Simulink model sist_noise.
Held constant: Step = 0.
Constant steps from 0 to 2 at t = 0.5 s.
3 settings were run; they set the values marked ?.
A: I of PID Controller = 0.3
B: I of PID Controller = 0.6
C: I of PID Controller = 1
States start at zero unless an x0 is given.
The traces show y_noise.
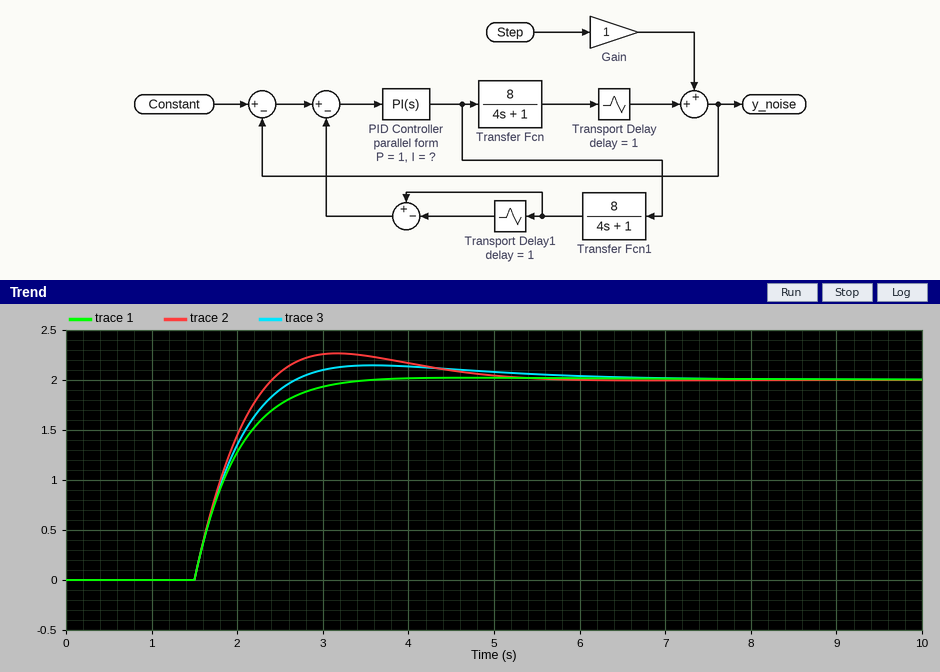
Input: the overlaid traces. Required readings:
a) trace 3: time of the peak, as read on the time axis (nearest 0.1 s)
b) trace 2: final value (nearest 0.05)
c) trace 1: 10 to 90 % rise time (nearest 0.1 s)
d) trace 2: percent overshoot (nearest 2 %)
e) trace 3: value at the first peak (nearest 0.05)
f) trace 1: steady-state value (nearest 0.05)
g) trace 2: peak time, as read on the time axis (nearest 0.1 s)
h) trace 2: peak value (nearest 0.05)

3.6 s
2.00
1.0 s
14 %
2.15
2.00
3.2 s
2.25
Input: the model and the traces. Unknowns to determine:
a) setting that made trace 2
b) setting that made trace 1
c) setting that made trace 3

C
A
B
